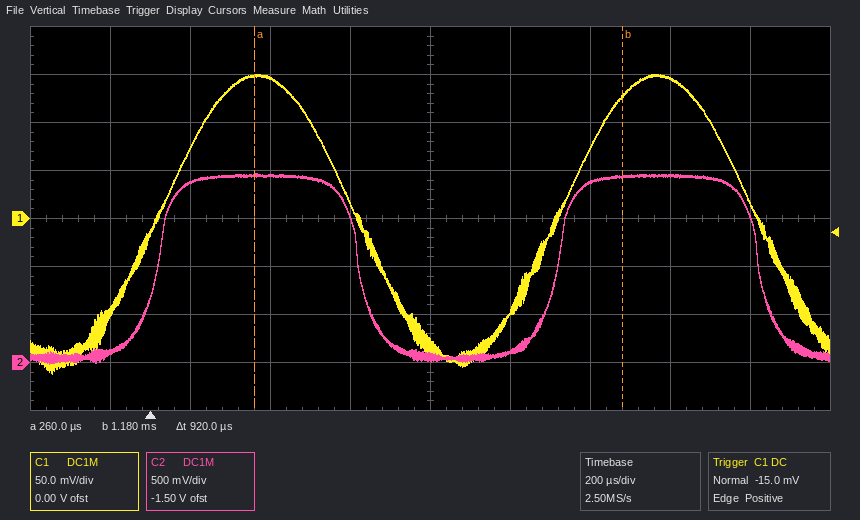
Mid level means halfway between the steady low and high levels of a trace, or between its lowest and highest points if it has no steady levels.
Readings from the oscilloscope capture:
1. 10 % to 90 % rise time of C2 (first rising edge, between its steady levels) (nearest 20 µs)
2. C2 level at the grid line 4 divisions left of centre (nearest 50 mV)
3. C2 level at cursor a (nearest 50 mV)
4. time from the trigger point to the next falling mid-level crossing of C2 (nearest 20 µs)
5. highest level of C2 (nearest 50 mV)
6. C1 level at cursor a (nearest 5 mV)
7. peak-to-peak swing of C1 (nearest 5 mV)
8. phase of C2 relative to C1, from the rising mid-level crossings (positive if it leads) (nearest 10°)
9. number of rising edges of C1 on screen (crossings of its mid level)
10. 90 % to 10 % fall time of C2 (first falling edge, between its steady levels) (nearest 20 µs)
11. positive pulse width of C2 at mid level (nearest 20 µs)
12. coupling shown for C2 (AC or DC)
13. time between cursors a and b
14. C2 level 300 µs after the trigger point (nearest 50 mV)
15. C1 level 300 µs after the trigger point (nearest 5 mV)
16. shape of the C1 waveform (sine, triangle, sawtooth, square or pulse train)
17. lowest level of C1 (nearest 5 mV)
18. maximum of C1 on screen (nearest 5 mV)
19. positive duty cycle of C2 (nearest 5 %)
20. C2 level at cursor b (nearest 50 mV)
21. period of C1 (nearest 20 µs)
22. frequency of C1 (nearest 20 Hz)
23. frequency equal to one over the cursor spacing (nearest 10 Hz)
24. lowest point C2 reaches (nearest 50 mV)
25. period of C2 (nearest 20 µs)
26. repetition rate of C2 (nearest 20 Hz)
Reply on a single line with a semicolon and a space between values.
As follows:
120 µs; 100 mV; 1.95 V; 520 µs; 1.95 V; 150 mV; 310 mV; 0°; 2; 120 µs; 500 µs; DC; 920 µs; 1.95 V; 145 mV; sine; -160 mV; 150 mV; 50 %; 1.95 V; 1.00 ms; 1.00 kHz; 1.09 kHz; 0 mV; 1.00 ms; 1.00 kHz
